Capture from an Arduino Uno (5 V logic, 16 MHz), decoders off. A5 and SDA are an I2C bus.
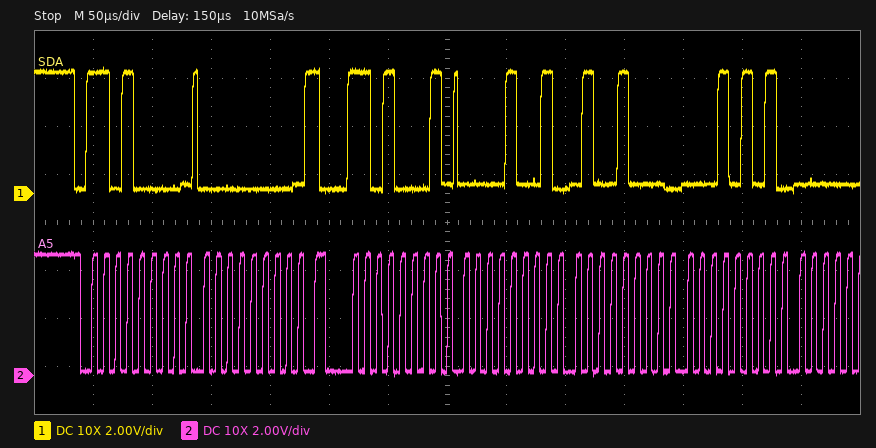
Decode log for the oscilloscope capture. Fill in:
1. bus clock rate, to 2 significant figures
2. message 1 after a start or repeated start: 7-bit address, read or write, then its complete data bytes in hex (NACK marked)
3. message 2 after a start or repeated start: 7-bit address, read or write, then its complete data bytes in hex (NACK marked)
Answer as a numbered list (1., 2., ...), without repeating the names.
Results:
1. 100 kHz
2. 0x68 write: 00
3. 0x68 read: 09 48 15
